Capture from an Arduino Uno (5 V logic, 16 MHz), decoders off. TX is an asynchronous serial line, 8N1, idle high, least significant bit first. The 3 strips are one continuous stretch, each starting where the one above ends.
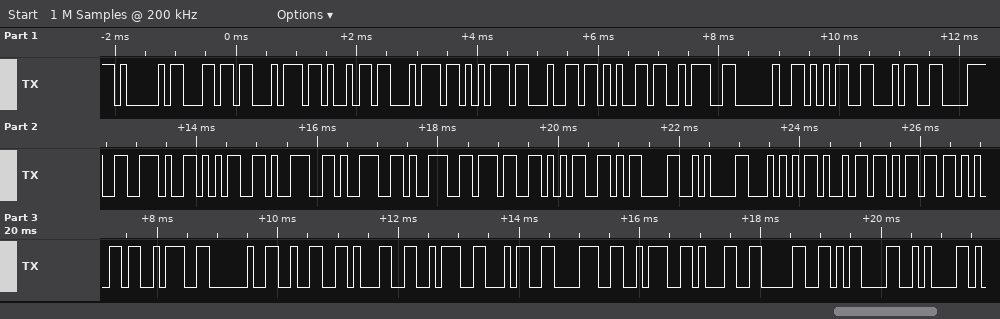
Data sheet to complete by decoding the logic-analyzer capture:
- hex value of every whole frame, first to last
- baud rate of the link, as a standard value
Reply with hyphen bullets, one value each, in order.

- 41 6C 74 69 74 75 64 65 3A 20 35 34 38 2E 35 39 39 39 37 35 0D 0A 54 69 6D 65 3A 20 32 31 3A 34 38 3A 31 30 0D 0A
- 9600 baud
